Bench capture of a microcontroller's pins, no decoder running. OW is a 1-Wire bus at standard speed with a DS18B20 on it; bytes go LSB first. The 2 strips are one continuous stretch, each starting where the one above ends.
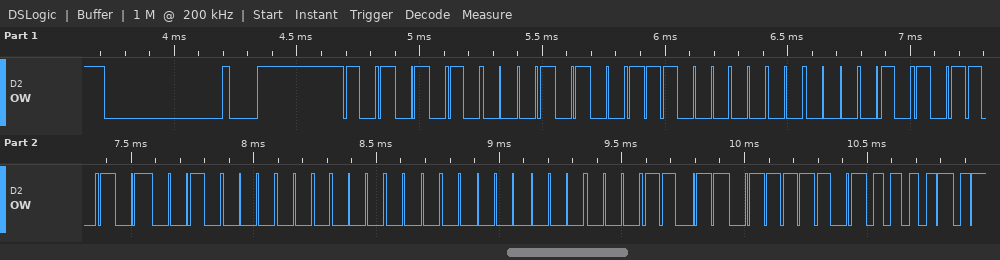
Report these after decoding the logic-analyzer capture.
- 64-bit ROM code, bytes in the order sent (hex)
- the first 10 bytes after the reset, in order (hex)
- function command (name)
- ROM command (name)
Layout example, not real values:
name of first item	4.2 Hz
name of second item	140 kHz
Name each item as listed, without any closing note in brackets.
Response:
64-bit ROM code, bytes in the order sent	28 07 40 AD 04 00 00 D8
the first 10 bytes after the reset, in order	55 28 07 40 AD 04 00 00 D8 BE
function command	Read Scratchpad
ROM command	Match ROM
